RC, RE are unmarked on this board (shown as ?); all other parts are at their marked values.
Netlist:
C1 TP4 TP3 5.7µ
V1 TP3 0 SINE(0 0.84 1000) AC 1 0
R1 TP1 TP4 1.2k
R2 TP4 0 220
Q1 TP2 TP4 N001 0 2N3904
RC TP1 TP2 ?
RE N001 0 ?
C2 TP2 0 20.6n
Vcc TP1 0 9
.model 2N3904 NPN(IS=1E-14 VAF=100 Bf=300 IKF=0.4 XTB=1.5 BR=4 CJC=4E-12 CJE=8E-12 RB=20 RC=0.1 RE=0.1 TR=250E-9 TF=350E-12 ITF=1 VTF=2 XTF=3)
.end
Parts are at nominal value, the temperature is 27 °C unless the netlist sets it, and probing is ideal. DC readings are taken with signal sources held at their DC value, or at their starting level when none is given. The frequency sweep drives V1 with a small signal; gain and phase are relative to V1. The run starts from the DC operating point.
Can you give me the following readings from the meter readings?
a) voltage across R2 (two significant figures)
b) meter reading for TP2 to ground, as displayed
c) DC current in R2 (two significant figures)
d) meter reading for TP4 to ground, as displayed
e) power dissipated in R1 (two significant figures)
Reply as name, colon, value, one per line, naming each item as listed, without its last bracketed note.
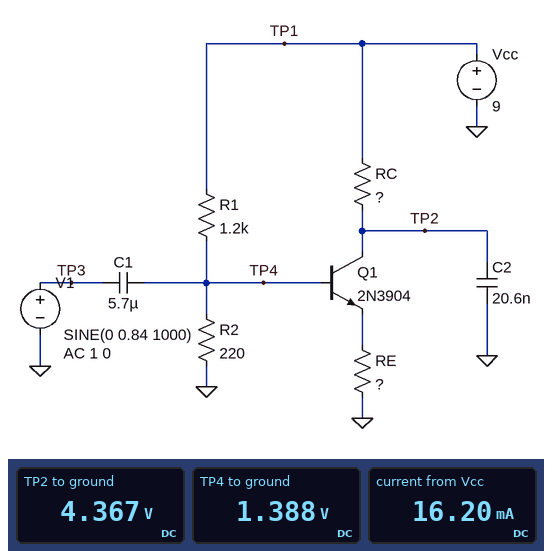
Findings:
voltage across R2: 1.4 V
meter reading for TP2 to ground, as displayed: 4.367 V
DC current in R2: 6.3 mA
meter reading for TP4 to ground, as displayed: 1.388 V
power dissipated in R1: 48 mW
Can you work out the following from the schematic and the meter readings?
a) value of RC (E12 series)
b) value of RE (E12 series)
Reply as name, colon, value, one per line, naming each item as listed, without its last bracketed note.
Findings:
value of RC: 470 Ω
value of RE: 68 Ω
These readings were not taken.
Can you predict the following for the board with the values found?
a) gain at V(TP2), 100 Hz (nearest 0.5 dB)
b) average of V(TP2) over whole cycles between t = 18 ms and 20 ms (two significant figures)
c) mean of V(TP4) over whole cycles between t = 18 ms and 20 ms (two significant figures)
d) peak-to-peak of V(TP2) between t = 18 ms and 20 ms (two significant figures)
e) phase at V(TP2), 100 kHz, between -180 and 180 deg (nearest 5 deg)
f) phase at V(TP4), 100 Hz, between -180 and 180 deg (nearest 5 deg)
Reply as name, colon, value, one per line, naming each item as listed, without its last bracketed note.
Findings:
gain at V(TP2), 100 Hz: 11.0 dB
average of V(TP2) over whole cycles between t = 18 ms and 20 ms: 5.0 V
mean of V(TP4) over whole cycles between t = 18 ms and 20 ms: 1.3 V
peak-to-peak of V(TP2) between t = 18 ms and 20 ms: 7.8 V
phase at V(TP2), 100 kHz, between -180 and 180 deg: 100 deg
phase at V(TP4), 100 Hz, between -180 and 180 deg: 55 deg
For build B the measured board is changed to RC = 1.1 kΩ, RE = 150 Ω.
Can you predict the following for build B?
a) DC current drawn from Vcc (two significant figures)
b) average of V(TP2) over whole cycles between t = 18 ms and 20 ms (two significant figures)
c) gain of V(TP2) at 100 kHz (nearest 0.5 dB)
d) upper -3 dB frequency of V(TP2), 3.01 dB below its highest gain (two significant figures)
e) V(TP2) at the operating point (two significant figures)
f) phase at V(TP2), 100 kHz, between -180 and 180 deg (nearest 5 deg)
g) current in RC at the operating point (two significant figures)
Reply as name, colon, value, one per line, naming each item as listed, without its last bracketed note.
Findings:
DC current drawn from Vcc: 11 mA
average of V(TP2) over whole cycles between t = 18 ms and 20 ms: 4.8 V
gain of V(TP2) at 100 kHz: -6.0 dB
upper -3 dB frequency of V(TP2), 3.01 dB below its highest gain: 7.3 kHz
V(TP2) at the operating point: 3.9 V
phase at V(TP2), 100 kHz, between -180 and 180 deg: 95 deg
current in RC at the operating point: 4.6 mA
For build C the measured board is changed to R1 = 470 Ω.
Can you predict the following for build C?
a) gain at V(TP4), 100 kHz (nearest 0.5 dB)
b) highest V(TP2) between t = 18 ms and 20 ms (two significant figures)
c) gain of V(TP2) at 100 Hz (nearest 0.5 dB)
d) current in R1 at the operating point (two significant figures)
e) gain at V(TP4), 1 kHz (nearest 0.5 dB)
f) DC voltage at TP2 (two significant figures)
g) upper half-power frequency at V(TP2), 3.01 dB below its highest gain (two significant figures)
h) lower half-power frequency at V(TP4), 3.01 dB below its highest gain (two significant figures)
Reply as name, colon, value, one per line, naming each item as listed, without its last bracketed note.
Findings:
gain at V(TP4), 100 kHz: 0 dB
highest V(TP2) between t = 18 ms and 20 ms: 4.5 V
gain of V(TP2) at 100 Hz: -18.0 dB
current in R1 at the operating point: 14 mA
gain at V(TP4), 1 kHz: -1.0 dB
DC voltage at TP2: 1.4 V
upper half-power frequency at V(TP2), 3.01 dB below its highest gain: 550 kHz
lower half-power frequency at V(TP4), 3.01 dB below its highest gain: 520 Hz
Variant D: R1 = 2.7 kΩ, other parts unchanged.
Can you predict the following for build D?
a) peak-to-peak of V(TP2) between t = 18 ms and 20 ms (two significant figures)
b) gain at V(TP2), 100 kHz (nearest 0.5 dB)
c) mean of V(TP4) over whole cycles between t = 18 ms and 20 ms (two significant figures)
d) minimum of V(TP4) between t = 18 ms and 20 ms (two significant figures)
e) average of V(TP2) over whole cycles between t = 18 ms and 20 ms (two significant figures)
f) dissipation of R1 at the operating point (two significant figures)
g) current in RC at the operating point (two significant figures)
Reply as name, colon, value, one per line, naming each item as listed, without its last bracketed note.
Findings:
peak-to-peak of V(TP2) between t = 18 ms and 20 ms: 5.4 V
gain at V(TP2), 100 kHz: -3.5 dB
mean of V(TP4) over whole cycles between t = 18 ms and 20 ms: 680 mV
minimum of V(TP4) between t = 18 ms and 20 ms: -160 mV
average of V(TP2) over whole cycles between t = 18 ms and 20 ms: 7.3 V
dissipation of R1 at the operating point: 26 mW
current in RC at the operating point: 570 µA
